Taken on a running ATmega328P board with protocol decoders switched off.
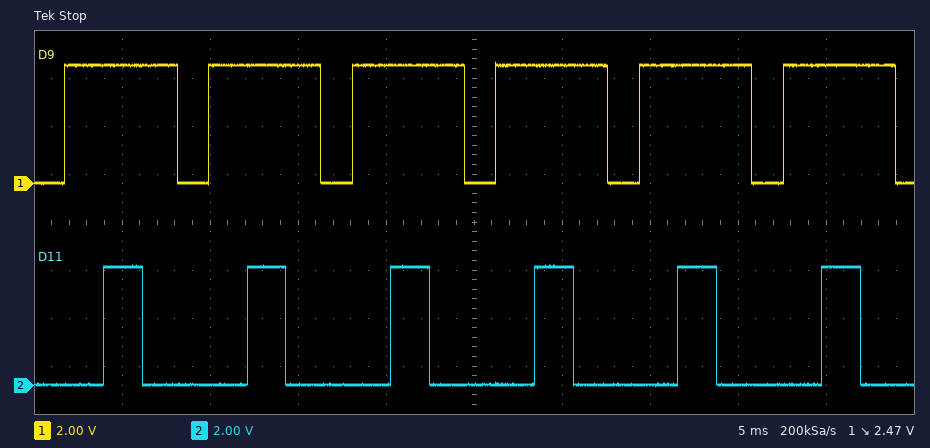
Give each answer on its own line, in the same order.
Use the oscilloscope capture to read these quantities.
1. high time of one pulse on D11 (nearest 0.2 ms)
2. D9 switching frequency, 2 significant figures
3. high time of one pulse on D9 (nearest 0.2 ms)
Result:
2.2 ms
120 Hz
6.4 ms
